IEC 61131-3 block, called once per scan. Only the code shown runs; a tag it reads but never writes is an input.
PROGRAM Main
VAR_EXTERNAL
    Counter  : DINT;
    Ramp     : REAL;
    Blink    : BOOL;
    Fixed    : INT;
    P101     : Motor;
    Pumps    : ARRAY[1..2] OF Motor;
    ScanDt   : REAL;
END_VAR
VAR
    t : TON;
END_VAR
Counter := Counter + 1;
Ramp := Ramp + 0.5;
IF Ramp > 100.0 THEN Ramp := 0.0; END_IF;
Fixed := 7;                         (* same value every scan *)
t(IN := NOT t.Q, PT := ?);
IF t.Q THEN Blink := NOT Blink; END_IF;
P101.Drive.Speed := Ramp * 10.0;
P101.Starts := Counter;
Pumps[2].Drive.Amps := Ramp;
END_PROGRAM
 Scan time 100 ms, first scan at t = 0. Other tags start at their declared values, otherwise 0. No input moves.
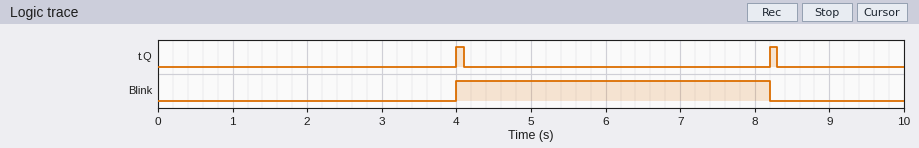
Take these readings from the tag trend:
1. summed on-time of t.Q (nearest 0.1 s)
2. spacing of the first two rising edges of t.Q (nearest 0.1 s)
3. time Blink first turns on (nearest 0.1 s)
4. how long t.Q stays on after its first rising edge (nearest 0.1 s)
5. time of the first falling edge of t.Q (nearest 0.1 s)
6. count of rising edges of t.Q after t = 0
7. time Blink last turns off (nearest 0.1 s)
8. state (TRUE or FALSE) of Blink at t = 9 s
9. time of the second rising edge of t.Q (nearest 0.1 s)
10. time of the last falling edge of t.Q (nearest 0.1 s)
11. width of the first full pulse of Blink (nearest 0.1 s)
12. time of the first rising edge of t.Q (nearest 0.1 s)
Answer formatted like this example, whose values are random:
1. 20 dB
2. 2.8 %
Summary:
1. 0.2 s
2. 4.2 s
3. 4.0 s
4. 0.1 s
5. 4.1 s
6. 2
7. 8.2 s
8. FALSE
9. 8.2 s
10. 8.3 s
11. 4.2 s
12. 4.0 s
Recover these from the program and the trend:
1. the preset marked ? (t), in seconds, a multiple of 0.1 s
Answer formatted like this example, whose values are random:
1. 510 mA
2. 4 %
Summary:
1. 4.0 s
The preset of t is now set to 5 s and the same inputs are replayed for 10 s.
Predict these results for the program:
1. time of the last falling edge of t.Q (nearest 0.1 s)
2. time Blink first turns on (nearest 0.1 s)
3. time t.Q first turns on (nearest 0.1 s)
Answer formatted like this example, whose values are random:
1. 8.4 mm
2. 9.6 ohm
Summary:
1. 5.1 s
2. 5.0 s
3. 5.0 s
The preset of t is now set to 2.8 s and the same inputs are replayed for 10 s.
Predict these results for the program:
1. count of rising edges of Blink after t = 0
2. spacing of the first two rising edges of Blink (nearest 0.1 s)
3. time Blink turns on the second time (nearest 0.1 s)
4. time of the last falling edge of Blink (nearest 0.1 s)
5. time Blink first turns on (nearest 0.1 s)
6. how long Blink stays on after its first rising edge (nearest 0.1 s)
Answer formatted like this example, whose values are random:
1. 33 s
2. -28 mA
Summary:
1. 2
2. 6.0 s
3. 8.8 s
4. 5.8 s
5. 2.8 s
6. 3.0 s
